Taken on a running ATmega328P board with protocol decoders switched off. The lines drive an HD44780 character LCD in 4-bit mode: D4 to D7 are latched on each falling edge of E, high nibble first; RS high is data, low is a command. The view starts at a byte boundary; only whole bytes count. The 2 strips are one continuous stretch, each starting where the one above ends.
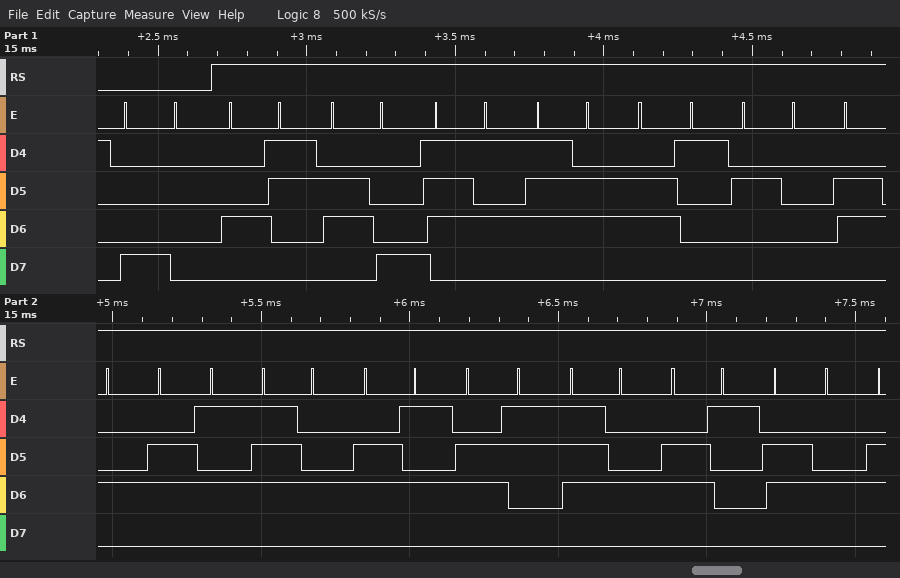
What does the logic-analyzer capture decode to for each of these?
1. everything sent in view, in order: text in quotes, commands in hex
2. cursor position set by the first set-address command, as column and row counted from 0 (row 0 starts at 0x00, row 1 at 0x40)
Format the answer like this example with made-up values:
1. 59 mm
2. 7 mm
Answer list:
1. 0x80 "Chuva detectad"
2. column 0, row 0
